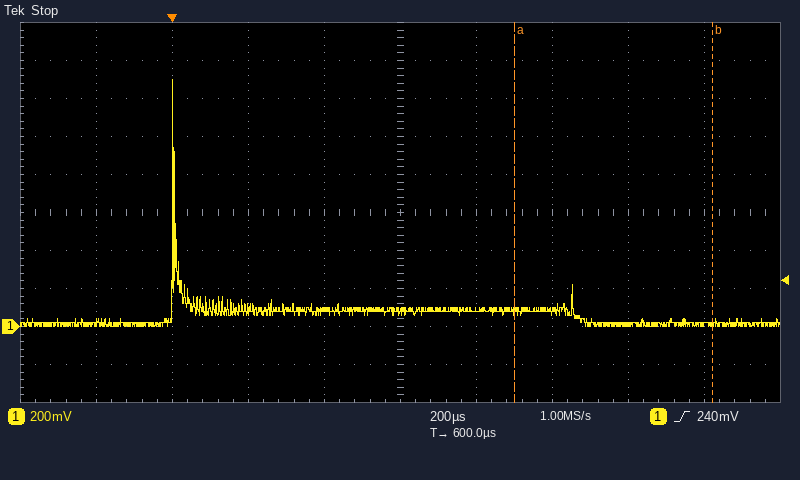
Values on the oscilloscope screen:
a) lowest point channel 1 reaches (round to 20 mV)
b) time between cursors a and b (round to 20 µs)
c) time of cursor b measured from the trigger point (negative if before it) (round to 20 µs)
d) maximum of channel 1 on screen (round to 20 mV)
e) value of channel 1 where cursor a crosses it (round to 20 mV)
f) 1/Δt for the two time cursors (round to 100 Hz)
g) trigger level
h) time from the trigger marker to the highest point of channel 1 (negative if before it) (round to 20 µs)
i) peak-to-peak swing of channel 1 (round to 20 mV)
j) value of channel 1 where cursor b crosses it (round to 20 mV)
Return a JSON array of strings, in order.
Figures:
["0 mV", "520 µs", "+1.42 ms", "1.30 V", "80 mV", "1.9 kHz", "240 mV", "0 µs", "1.30 V", "20 mV"]
